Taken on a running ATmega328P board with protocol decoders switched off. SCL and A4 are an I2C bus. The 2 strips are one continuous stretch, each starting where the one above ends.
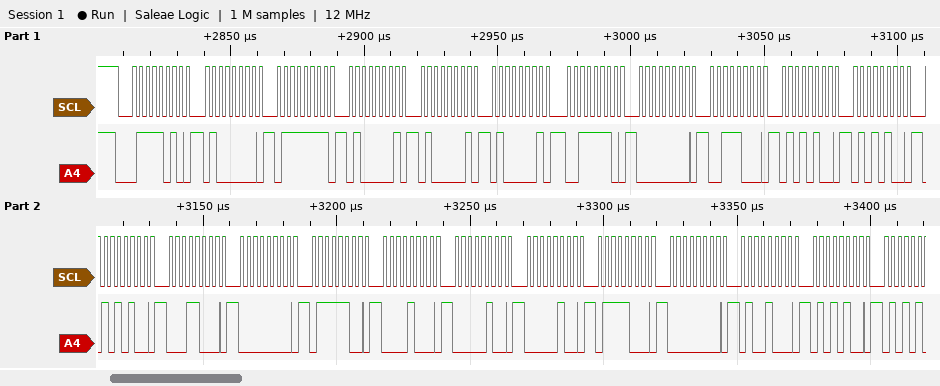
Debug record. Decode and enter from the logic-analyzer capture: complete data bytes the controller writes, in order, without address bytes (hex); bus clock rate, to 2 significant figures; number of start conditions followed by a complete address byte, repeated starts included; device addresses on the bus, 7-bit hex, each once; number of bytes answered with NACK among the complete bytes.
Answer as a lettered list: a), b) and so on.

a) 40 7F 41 41 41 3E 00 38 54 54 54 18 00 7C 08 04 04 78 00 48 54
b) 400 kHz
c) 1
d) 0x3D
e) 0
